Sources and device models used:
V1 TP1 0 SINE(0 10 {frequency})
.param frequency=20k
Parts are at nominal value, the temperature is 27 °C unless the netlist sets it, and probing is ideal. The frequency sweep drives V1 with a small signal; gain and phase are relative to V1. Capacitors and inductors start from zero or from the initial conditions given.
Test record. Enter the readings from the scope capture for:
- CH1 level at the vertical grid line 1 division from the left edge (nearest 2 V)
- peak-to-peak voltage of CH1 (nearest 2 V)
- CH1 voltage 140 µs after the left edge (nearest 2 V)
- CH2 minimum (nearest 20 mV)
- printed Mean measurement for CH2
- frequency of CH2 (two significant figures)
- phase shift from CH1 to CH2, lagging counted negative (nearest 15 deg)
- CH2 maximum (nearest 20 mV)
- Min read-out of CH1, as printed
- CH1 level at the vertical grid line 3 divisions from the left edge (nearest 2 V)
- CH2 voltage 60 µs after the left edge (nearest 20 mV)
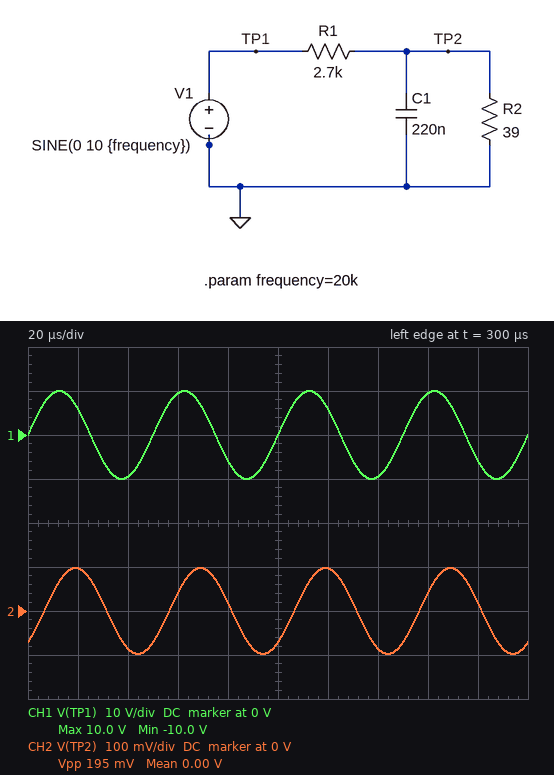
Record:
6 V
20 V
-10 V
-100 mV
0.00 V
20 kHz
-45 deg
100 mV
-10.0 V
10 V
40 mV
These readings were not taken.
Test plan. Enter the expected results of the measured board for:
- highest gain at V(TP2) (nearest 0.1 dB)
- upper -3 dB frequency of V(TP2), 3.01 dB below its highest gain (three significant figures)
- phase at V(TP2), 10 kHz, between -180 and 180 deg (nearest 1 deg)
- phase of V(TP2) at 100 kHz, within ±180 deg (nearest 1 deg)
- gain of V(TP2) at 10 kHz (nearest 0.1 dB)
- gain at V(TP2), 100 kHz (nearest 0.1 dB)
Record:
-36.9 dB
18.8 kHz
-28 deg
-79 deg
-38.0 dB
-51.6 dB
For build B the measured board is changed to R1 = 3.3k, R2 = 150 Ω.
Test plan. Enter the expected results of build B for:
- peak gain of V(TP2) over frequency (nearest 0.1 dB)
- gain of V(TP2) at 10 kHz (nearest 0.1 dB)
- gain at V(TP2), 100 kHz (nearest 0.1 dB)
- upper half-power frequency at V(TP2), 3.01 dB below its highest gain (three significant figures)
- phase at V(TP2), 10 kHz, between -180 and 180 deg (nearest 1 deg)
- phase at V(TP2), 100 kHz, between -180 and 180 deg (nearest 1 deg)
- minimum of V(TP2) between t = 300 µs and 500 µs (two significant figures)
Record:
-27.2 dB
-34.2 dB
-53.2 dB
5.04 kHz
-63 deg
-87 deg
-110 mV
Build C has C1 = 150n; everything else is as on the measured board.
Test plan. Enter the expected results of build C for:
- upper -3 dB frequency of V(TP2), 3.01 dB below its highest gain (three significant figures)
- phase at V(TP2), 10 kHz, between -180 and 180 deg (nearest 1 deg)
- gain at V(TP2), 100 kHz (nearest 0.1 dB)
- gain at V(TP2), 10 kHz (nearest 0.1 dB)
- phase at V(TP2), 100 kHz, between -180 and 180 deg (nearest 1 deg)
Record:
27.6 kHz
-20 deg
-48.4 dB
-37.5 dB
-75 deg
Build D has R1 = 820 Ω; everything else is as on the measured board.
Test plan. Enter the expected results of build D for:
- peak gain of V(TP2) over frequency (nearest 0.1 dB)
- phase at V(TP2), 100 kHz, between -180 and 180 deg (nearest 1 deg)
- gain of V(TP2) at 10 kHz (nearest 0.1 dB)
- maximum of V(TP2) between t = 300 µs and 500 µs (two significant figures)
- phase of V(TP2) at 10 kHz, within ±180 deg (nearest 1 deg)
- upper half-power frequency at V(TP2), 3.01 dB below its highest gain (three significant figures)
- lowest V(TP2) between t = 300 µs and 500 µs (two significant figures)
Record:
-26.9 dB
-79 deg
-27.9 dB
320 mV
-27 deg
19.4 kHz
-320 mV
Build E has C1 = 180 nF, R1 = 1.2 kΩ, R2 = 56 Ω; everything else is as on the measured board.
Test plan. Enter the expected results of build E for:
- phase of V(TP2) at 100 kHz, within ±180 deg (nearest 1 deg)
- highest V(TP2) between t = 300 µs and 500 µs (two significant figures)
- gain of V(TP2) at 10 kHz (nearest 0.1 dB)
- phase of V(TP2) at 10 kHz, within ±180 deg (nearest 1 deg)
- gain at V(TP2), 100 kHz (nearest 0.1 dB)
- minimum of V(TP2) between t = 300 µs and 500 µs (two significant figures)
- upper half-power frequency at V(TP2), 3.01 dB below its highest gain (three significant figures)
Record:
-81 deg
280 mV
-28.4 dB
-31 deg
-42.8 dB
-280 mV
16.5 kHz
